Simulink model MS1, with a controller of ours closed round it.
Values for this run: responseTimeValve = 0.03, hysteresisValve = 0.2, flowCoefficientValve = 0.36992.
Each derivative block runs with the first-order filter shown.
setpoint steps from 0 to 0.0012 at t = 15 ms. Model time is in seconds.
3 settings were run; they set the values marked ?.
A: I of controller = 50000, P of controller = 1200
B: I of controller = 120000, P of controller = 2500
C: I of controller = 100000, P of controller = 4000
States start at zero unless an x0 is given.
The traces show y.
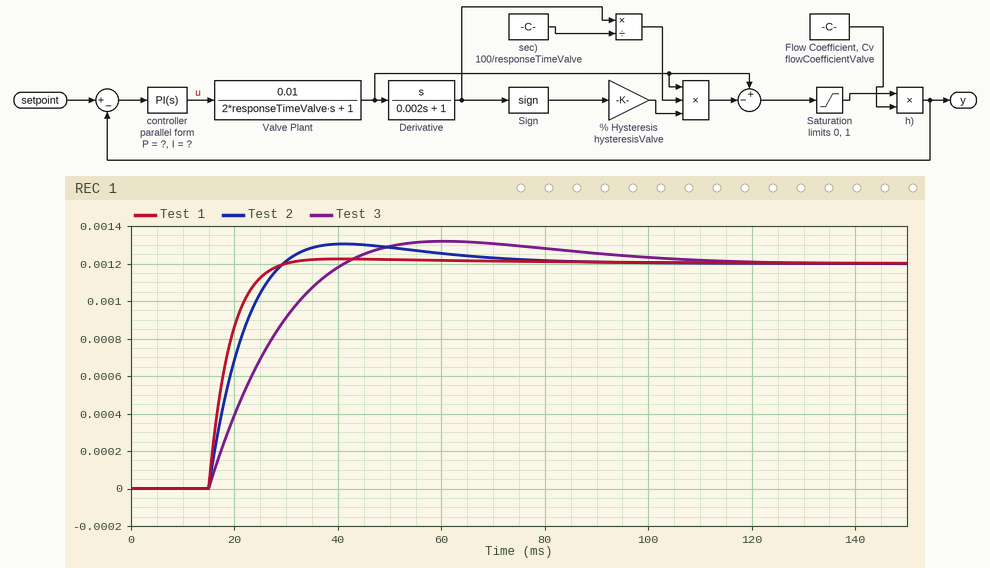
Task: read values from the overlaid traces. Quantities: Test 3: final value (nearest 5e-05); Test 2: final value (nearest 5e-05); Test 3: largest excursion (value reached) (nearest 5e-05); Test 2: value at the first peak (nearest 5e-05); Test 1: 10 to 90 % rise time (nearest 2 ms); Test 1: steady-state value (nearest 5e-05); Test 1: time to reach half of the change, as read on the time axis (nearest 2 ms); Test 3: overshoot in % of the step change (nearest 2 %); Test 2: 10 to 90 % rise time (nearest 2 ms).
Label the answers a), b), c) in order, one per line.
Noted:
a) 0.00120
b) 0.00120
c) 0.00130
d) 0.00130
e) 8 ms
f) 0.00120
g) 18 ms
h) 10 %
i) 10 ms
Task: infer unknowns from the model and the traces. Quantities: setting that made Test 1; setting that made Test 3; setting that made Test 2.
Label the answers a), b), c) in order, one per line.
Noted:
a) C
b) A
c) B
